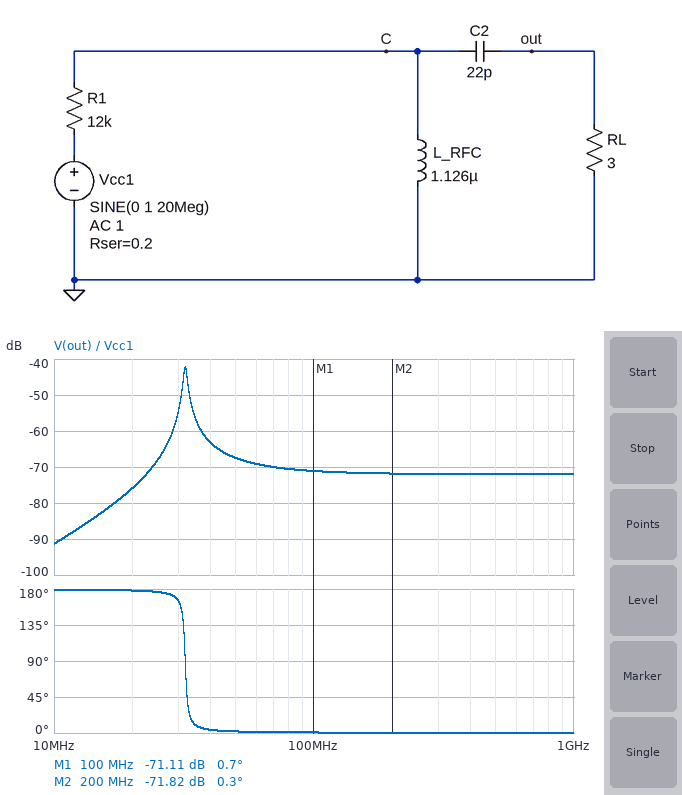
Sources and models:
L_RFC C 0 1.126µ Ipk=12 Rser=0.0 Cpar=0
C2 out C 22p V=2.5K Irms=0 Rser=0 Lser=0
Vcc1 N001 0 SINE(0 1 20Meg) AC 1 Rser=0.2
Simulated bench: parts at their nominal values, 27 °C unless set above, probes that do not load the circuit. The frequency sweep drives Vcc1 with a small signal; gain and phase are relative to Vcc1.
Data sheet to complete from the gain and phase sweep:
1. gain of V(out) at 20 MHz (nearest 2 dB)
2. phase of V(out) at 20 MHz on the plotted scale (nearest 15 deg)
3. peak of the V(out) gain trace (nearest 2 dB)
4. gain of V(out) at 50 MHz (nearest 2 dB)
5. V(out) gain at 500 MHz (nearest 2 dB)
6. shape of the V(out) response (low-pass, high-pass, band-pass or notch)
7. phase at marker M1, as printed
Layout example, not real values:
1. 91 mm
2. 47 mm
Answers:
1. -76 dB
2. 180 deg
3. -42 dB
4. -68 dB
5. -72 dB
6. high-pass
7. 0.7 deg
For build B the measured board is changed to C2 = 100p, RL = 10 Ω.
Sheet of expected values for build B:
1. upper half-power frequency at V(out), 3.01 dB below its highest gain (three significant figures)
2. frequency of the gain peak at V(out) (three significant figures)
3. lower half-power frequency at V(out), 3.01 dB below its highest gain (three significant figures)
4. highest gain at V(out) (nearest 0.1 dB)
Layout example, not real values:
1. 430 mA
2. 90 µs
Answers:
1. 15.9 MHz
2. 15.0 MHz
3. 14.3 MHz
4. -41.8 dB
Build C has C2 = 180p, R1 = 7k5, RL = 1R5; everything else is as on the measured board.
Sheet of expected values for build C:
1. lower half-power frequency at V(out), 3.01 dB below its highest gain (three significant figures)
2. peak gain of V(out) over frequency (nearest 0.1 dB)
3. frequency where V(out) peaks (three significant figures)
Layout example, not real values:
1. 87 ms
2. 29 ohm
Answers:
1. 11.0 MHz
2. -43.4 dB
3. 11.2 MHz
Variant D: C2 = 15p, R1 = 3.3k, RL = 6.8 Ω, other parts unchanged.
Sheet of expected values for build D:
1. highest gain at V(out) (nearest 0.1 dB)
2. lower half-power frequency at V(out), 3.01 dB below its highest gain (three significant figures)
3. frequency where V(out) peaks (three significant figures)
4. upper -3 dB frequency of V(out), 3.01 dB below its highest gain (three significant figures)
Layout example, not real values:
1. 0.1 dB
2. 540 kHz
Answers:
1. -34.4 dB
2. 36.9 MHz
3. 38.8 MHz
4. 41.1 MHz
